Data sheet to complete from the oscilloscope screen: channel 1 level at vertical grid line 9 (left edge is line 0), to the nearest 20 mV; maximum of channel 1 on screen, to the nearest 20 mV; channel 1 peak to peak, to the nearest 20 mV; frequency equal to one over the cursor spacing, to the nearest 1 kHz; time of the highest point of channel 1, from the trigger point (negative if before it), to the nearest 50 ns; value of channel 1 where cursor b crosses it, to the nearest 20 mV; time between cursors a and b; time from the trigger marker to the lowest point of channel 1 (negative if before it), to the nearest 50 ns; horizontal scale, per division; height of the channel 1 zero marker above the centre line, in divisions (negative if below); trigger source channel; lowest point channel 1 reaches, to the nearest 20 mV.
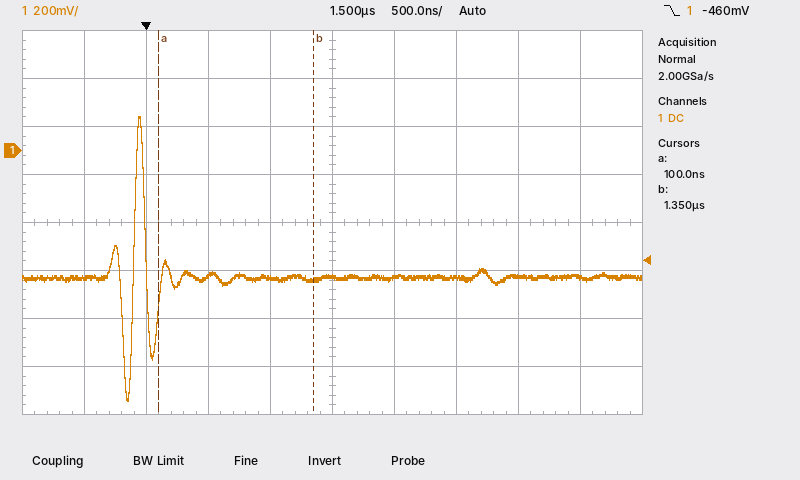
-520 mV
140 mV
1.18 V
800 kHz
-50 ns
-540 mV
1.25 µs
-150 ns
500 ns
+1.5 div
channel 1
-1.04 V
